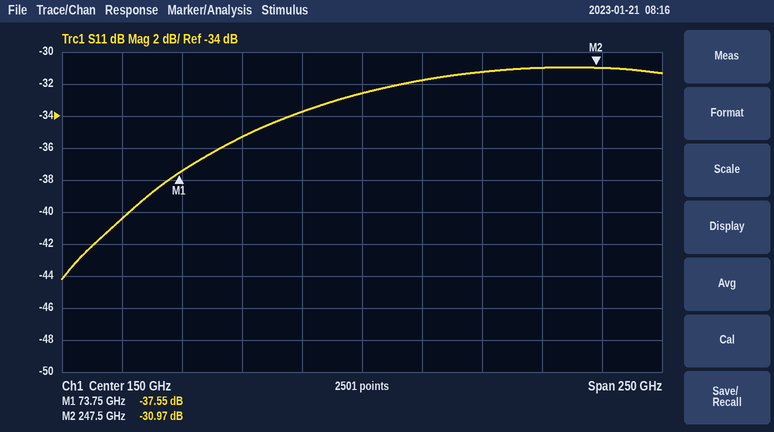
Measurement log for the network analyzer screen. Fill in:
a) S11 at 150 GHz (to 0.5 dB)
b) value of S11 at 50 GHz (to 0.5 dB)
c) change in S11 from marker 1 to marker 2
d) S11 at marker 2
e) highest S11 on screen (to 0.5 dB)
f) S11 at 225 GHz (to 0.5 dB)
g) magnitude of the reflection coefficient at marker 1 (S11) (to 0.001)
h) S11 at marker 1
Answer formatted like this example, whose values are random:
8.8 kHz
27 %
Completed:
-32.5 dB
-40.5 dB
6.58 dB
-30.97 dB
-31.0 dB
-31.0 dB
0.013
-37.55 dB
